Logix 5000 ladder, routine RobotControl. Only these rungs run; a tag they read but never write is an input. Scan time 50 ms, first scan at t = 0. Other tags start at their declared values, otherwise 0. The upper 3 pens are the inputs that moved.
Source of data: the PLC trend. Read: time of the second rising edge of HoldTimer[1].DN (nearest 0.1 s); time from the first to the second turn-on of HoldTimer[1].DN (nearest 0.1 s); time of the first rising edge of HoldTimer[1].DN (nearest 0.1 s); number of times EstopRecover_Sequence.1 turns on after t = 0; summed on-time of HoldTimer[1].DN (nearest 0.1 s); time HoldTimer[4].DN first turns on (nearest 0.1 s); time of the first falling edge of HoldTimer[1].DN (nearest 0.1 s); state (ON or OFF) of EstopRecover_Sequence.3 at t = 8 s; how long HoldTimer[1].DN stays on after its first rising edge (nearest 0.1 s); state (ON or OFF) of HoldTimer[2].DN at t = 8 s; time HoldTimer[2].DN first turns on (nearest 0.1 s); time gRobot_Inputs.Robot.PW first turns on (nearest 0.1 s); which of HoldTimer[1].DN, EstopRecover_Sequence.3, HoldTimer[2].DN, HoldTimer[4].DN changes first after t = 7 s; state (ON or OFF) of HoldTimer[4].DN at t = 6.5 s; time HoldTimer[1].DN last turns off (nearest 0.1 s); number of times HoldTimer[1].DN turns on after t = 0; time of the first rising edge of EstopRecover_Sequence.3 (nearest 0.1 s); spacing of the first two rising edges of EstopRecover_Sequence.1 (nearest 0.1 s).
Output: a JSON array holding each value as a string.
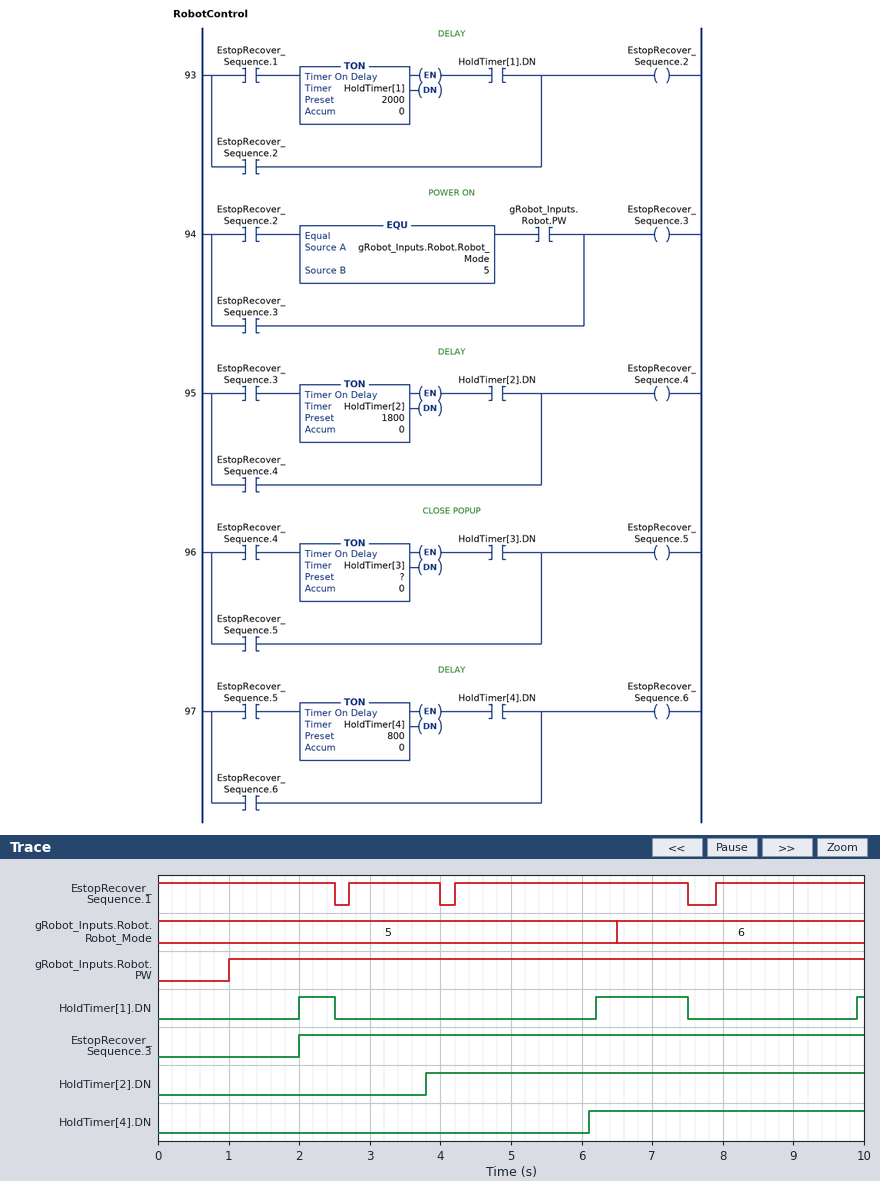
["6.2 s", "4.2 s", "2.0 s", "3", "1.9 s", "6.1 s", "2.5 s", "ON", "0.5 s", "ON", "3.8 s", "1.0 s", "HoldTimer[1].DN", "ON", "7.5 s", "3", "2.0 s", "1.5 s"]
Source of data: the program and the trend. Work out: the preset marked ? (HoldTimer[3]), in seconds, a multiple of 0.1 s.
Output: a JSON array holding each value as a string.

["1.5 s"]
